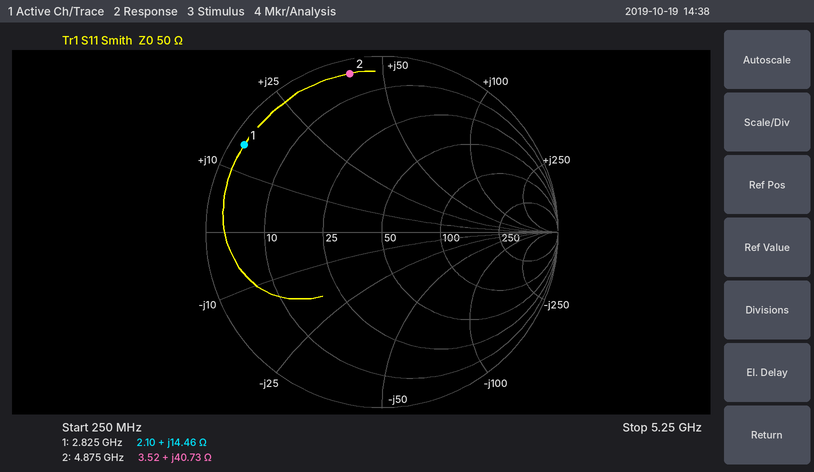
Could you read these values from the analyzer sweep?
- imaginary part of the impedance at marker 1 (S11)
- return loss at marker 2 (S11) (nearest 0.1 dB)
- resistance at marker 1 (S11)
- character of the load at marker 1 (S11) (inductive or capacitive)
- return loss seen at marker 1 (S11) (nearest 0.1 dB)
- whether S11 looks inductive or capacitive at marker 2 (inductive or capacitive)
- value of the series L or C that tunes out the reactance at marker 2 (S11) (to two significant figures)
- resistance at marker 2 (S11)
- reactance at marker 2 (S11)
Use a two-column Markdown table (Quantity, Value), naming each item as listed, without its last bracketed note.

| Quantity | Value |
|---|---|
| imaginary part of the impedance at marker 1 | +14.46 Ω |
| return loss at marker 2 (S11) | 0.7 dB |
| resistance at marker 1 | 2.10 Ω |
| character of the load at marker 1 (S11) | inductive |
| return loss seen at marker 1 (S11) | 0.7 dB |
| whether S11 looks inductive or capacitive at marker 2 | inductive |
| value of the series L or C that tunes out the reactance at marker 2 (S11) | 800 fF |
| resistance at marker 2 | 3.52 Ω |
| reactance at marker 2 | +40.73 Ω |
